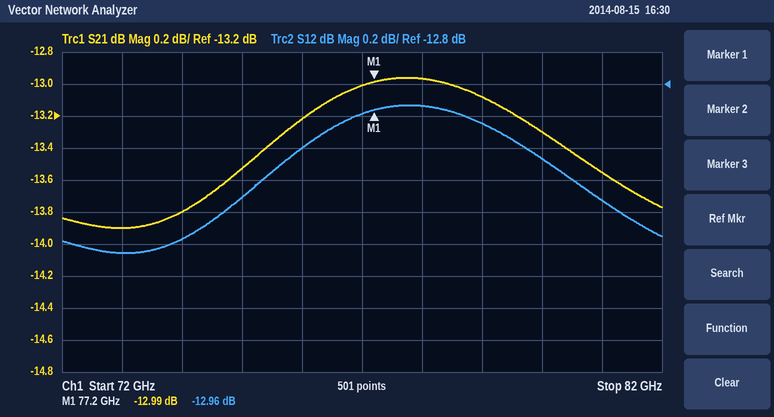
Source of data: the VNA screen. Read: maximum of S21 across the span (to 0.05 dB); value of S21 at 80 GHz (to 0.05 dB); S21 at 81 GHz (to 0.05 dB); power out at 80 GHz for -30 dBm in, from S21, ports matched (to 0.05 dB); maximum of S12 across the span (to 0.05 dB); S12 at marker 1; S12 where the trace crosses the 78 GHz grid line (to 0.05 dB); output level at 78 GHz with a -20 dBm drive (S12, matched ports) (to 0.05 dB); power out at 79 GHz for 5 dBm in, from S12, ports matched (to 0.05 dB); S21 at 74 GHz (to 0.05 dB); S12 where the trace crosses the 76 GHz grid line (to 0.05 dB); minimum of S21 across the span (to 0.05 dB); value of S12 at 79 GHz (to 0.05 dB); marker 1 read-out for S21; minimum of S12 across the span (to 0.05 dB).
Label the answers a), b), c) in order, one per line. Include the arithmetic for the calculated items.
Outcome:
a) -12.95 dB
b) -13.30 dB
c) -13.55 dB
d) -30 dBm + (-13.30 dB) = -43.30 dBm
e) -12.95 dB
f) -12.96 dB
g) -12.95 dB
h) -20 dBm + (-12.95 dB) = -32.95 dBm
i) 5 dBm + (-13.05 dB) = -8.05 dBm
j) -13.80 dB
k) -13.20 dB
l) -13.90 dB
m) -13.05 dB
n) -12.99 dB
o) -13.85 dB
